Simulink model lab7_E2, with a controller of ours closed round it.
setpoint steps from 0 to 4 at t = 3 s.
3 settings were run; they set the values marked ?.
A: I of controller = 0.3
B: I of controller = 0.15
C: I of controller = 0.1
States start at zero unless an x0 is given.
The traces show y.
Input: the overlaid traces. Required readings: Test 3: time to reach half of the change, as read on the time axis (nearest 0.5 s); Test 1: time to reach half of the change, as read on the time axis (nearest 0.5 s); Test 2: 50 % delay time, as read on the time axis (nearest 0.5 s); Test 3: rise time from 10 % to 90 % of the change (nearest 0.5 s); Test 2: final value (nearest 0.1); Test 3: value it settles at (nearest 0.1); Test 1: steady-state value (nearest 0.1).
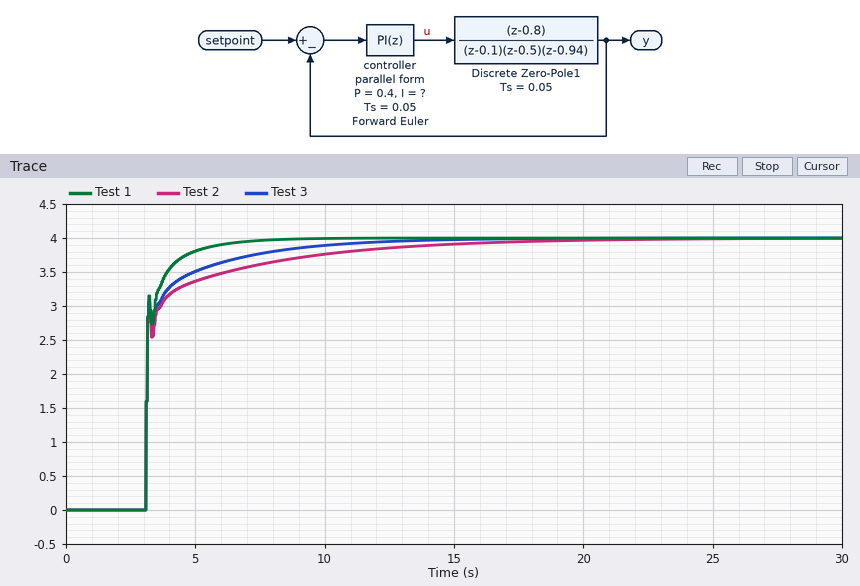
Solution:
3.0 s
3.0 s
3.0 s
2.5 s
4.0
4.0
4.0
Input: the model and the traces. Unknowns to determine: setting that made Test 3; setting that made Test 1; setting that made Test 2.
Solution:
B
A
C
